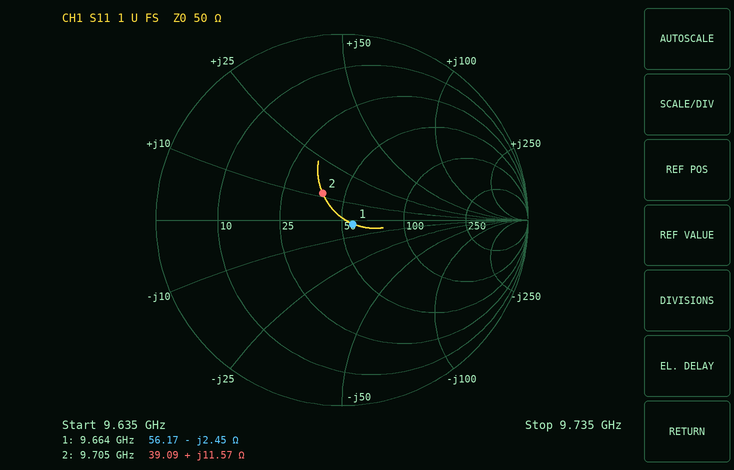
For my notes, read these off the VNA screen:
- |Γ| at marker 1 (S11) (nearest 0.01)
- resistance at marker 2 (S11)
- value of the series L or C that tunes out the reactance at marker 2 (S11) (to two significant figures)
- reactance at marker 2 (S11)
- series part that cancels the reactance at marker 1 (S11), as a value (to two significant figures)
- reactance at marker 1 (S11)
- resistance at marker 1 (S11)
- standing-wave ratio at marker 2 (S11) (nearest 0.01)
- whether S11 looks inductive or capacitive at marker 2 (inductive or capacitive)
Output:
0.06
39.09 Ω
1.4 pF
+11.57 Ω
40 pH
-2.45 Ω
56.17 Ω
1.43
inductive
